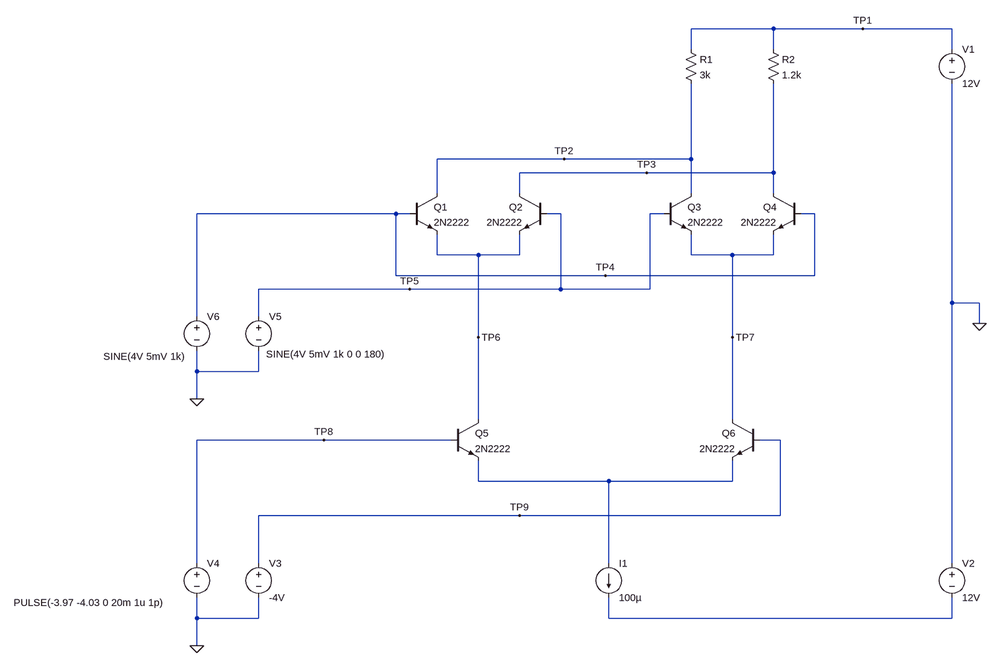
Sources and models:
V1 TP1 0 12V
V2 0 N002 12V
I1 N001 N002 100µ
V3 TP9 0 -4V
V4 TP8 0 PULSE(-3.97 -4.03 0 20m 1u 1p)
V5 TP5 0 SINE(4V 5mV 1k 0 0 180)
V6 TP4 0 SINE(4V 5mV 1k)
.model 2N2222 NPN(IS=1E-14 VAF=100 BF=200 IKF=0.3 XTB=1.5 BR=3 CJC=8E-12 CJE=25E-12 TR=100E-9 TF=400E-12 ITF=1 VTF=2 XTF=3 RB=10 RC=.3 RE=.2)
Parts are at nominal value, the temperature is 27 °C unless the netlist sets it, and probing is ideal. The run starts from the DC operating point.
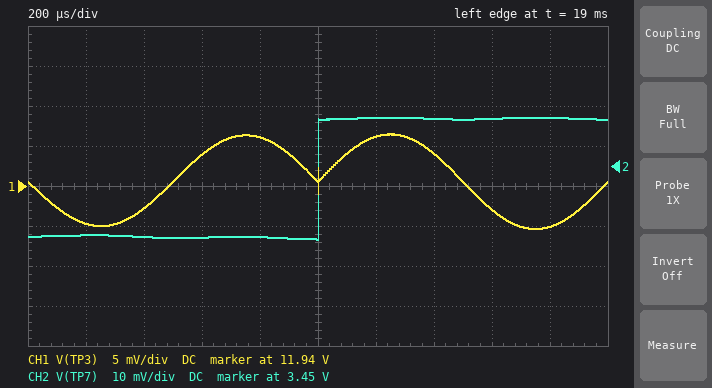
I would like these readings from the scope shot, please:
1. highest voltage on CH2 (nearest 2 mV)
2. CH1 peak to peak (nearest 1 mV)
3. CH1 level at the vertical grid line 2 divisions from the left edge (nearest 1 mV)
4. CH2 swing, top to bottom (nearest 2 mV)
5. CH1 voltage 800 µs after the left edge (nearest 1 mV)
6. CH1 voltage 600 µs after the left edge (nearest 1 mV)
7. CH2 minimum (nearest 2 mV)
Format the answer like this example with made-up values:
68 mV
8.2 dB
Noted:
3.462 V
12 mV
11.937 V
30 mV
11.946 V
11.944 V
3.432 V
